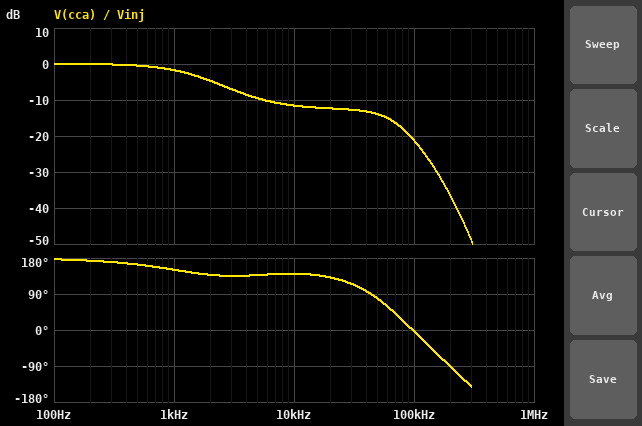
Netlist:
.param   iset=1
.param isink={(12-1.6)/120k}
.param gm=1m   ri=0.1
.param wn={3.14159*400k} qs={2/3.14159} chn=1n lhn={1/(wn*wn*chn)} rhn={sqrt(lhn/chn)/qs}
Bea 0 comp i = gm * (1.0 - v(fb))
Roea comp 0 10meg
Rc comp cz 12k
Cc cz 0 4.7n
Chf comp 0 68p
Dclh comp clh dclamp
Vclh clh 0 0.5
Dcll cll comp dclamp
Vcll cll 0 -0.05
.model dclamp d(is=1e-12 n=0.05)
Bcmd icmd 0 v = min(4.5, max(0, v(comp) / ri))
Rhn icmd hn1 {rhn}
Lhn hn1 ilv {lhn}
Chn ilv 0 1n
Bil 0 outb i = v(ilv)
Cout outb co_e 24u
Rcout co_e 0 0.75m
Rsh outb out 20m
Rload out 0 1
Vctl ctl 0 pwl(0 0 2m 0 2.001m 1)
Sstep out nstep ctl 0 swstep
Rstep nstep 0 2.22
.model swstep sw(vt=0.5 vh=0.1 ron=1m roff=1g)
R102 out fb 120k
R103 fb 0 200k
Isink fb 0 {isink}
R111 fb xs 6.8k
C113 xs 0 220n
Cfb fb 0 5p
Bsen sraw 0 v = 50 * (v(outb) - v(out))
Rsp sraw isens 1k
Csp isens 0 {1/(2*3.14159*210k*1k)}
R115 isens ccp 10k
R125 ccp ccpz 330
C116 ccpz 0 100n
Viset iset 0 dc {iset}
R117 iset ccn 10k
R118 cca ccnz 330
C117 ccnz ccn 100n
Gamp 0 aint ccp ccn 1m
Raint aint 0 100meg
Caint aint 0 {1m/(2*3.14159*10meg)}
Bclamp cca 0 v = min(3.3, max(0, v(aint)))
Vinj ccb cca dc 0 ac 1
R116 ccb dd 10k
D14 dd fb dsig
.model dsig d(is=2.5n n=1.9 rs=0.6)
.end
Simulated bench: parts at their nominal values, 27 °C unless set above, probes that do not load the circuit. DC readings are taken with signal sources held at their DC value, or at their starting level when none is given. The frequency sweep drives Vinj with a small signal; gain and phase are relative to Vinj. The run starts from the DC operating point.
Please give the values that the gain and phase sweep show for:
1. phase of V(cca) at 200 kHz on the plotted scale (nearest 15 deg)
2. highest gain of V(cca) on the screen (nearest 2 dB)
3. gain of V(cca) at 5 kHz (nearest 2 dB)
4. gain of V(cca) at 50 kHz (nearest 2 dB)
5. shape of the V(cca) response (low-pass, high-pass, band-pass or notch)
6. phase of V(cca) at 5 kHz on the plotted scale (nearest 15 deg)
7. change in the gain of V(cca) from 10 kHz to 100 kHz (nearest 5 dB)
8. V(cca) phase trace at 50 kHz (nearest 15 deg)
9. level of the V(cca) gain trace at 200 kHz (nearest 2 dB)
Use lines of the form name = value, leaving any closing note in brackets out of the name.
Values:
phase of V(cca) at 200 kHz on the plotted scale = -90 deg
highest gain of V(cca) on the screen = 0 dB
gain of V(cca) at 5 kHz = -10 dB
gain of V(cca) at 50 kHz = -14 dB
shape of the V(cca) response = low-pass
phase of V(cca) at 5 kHz on the plotted scale = 135 deg
change in the gain of V(cca) from 10 kHz to 100 kHz = -10 dB
V(cca) phase trace at 50 kHz = 75 deg
level of the V(cca) gain trace at 200 kHz = -36 dB
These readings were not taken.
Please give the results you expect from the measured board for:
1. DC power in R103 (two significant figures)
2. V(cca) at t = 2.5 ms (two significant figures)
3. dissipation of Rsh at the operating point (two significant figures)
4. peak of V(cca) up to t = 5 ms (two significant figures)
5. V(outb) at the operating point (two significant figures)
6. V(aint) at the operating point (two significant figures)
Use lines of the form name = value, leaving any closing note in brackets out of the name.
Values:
DC power in R103 = 5.0 µW
V(cca) at t = 2.5 ms = 2.5 V
dissipation of Rsh at the operating point = 20 mW
peak of V(cca) up to t = 5 ms = 2.5 V
V(outb) at the operating point = 1.0 V
V(aint) at the operating point = 2.4 V
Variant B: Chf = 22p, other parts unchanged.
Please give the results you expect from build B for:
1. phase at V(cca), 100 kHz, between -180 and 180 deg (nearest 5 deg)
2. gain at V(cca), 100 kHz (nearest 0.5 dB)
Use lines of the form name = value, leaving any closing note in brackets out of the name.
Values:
phase at V(cca), 100 kHz, between -180 and 180 deg = 20 deg
gain at V(cca), 100 kHz = -20.5 dB
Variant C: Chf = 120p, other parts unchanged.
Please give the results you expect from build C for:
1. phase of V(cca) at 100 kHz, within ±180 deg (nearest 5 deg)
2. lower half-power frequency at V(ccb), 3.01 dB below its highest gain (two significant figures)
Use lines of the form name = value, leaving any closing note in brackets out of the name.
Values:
phase of V(cca) at 100 kHz, within ±180 deg = -25 deg
lower half-power frequency at V(ccb), 3.01 dB below its highest gain = 8.5 kHz
